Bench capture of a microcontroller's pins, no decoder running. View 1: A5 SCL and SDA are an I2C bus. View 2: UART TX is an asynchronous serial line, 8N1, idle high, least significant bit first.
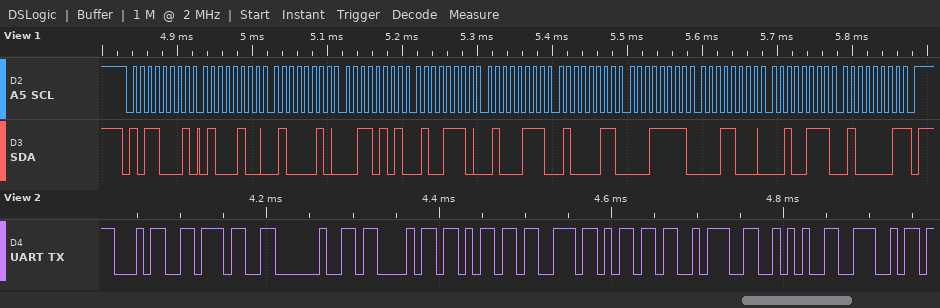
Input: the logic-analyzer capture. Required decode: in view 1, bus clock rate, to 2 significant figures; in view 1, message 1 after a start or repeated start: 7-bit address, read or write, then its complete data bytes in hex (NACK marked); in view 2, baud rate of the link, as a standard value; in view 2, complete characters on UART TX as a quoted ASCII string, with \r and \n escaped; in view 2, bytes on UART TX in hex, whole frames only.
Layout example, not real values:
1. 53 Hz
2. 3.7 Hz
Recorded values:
1. 100 kHz
2. 0x58 read: 44 42 35 4E 47 43 1F 18 27 41 NACK
3. 115200 baud
4. "47 Cksm:*N"
5. 34 37 20 43 6B 73 6D 3A 2A 4E
